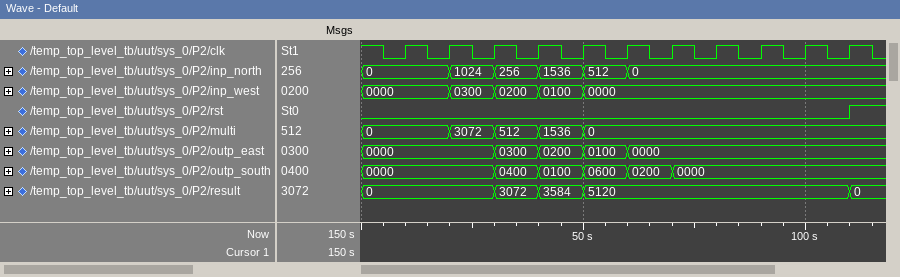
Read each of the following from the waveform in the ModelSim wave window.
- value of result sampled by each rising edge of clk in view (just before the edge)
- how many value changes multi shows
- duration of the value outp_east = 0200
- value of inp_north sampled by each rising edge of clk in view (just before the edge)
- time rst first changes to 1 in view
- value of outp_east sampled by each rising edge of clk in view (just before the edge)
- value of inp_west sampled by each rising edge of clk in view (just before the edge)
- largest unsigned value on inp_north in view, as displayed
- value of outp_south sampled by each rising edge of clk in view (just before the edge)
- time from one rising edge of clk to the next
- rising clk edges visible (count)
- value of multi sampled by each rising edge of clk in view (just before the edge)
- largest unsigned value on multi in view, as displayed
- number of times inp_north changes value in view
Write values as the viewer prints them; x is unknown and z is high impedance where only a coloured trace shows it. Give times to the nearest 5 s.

0, 0, 0, 3072, 3584, 5120, 5120, 5120, 5120, 5120, 5120
4
10 s
0, 0, 1024, 256, 1536, 512, 0, 0, 0, 0, 0
110 s
0000, 0000, 0000, 0300, 0200, 0100, 0000, 0000, 0000, 0000, 0000
0000, 0000, 0300, 0200, 0100, 0000, 0000, 0000, 0000, 0000, 0000
1536
0000, 0000, 0000, 0400, 0100, 0600, 0200, 0000, 0000, 0000, 0000
10 s
11
0, 0, 3072, 512, 1536, 0, 0, 0, 0, 0, 0
3072
5
